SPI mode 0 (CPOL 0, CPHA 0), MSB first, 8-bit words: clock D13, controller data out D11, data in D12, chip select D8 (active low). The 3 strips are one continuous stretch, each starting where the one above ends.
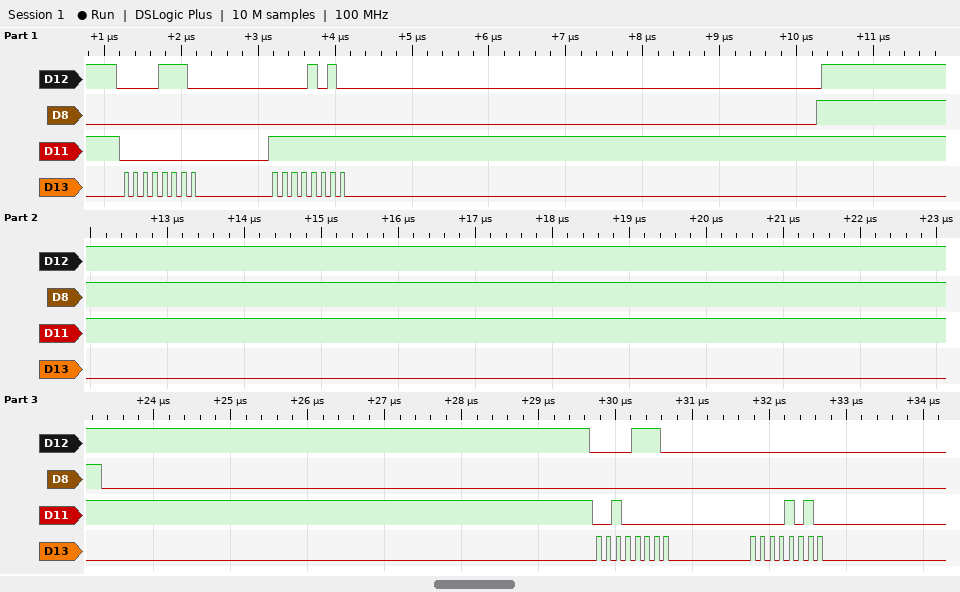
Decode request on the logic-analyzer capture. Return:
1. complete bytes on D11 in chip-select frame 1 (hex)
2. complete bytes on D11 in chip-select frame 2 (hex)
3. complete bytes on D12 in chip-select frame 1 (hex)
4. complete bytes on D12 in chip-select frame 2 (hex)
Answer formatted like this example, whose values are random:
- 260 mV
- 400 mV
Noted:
- 0x00 0xFF
- 0x20 0x0A
- 0x0E 0x0A
- 0x0E 0x00
